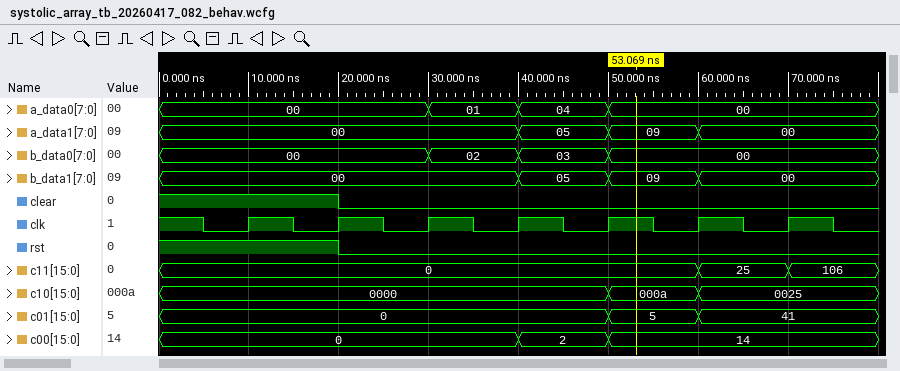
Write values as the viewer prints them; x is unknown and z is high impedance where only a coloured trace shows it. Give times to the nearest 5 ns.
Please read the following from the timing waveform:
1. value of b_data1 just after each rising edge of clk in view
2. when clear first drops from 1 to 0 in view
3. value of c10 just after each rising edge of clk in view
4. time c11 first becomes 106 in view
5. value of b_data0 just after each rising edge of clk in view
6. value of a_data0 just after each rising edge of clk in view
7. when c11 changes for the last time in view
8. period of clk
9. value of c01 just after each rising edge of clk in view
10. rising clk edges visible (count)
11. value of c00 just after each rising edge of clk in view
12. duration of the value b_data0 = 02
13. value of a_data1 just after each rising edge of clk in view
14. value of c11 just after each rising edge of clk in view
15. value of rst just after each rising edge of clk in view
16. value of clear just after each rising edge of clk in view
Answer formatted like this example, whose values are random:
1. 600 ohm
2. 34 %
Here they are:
1. 00, 00, 00, 05, 09, 00, 00
2. 20 ns
3. 0000, 0000, 0000, 0000, 000a, 0025, 0025
4. 70 ns
5. 00, 00, 02, 03, 00, 00, 00
6. 00, 00, 01, 04, 00, 00, 00
7. 70 ns
8. 10 ns
9. 0, 0, 0, 0, 5, 41, 41
10. 7
11. 0, 0, 0, 2, 14, 14, 14
12. 10 ns
13. 00, 00, 00, 05, 09, 00, 00
14. 0, 0, 0, 0, 0, 25, 106
15. 1 0 0 0 0 0 0
16. 1 0 0 0 0 0 0
